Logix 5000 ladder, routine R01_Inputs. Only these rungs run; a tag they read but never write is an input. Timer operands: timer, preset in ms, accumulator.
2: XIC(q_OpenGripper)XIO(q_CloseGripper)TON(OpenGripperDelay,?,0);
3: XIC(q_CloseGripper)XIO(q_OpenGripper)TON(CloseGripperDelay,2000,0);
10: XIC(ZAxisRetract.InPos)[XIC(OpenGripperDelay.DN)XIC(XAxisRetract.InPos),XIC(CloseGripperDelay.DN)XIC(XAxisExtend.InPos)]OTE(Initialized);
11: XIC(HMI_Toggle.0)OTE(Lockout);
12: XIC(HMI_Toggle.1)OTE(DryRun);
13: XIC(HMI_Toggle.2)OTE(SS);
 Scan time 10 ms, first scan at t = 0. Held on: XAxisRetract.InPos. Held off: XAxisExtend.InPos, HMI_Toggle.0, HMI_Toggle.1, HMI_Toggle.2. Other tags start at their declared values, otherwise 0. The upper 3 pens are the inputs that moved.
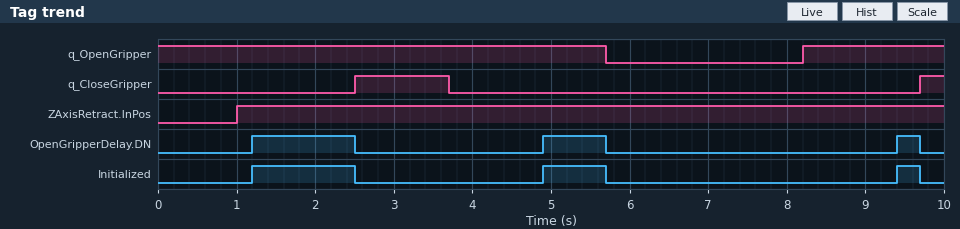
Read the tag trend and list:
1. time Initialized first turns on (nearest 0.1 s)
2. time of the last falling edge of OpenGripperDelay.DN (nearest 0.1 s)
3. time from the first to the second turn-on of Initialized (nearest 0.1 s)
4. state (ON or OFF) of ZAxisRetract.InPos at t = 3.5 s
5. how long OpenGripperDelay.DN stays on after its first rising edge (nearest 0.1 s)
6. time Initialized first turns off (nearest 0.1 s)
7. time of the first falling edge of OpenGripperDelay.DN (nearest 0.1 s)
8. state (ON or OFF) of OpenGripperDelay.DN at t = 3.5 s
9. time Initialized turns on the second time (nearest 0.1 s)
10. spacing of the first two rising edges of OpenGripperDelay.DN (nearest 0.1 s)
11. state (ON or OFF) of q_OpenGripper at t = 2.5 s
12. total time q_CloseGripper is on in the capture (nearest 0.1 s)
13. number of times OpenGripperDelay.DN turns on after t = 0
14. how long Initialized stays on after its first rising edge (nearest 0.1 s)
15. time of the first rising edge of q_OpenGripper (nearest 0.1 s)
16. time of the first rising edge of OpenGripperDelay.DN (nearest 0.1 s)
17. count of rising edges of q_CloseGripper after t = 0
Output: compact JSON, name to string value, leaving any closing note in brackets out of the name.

{"time Initialized first turns on": "1.2 s", "time of the last falling edge of OpenGripperDelay.DN": "9.7 s", "time from the first to the second turn-on of Initialized": "3.7 s", "state (ON or OFF) of ZAxisRetract.InPos at t = 3.5 s": "ON", "how long OpenGripperDelay.DN stays on after its first rising edge": "1.3 s", "time Initialized first turns off": "2.5 s", "time of the first falling edge of OpenGripperDelay.DN": "2.5 s", "state (ON or OFF) of OpenGripperDelay.DN at t = 3.5 s": "OFF", "time Initialized turns on the second time": "4.9 s", "spacing of the first two rising edges of OpenGripperDelay.DN": "3.7 s", "state (ON or OFF) of q_OpenGripper at t = 2.5 s": "ON", "total time q_CloseGripper is on in the capture": "1.5 s", "number of times OpenGripperDelay.DN turns on after t = 0": "3", "how long Initialized stays on after its first rising edge": "1.3 s", "time of the first rising edge of q_OpenGripper": "8.2 s", "time of the first rising edge of OpenGripperDelay.DN": "1.2 s", "count of rising edges of q_CloseGripper after t = 0": "2"}
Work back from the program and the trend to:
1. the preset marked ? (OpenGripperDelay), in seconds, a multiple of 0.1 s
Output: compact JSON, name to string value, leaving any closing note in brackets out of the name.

{"the preset marked ? (OpenGripperDelay), in seconds, a multiple of 0.1 s": "1.2 s"}
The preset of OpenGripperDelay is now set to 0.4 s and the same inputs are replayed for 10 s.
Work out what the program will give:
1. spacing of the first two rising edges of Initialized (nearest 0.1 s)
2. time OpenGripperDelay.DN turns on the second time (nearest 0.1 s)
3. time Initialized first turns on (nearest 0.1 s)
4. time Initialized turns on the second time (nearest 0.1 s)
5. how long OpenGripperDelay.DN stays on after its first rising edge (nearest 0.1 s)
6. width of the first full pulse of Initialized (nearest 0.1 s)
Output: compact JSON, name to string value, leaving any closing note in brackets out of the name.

{"spacing of the first two rising edges of Initialized": "3.1 s", "time OpenGripperDelay.DN turns on the second time": "4.1 s", "time Initialized first turns on": "1.0 s", "time Initialized turns on the second time": "4.1 s", "how long OpenGripperDelay.DN stays on after its first rising edge": "2.1 s", "width of the first full pulse of Initialized": "1.5 s"}
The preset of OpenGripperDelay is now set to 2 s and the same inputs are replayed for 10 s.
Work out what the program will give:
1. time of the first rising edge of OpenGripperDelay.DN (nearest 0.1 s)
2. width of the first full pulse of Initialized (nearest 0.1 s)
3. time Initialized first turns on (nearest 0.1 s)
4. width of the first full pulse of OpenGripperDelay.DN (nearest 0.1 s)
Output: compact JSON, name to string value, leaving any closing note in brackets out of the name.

{"time of the first rising edge of OpenGripperDelay.DN": "2.0 s", "width of the first full pulse of Initialized": "0.5 s", "time Initialized first turns on": "2.0 s", "width of the first full pulse of OpenGripperDelay.DN": "0.5 s"}
